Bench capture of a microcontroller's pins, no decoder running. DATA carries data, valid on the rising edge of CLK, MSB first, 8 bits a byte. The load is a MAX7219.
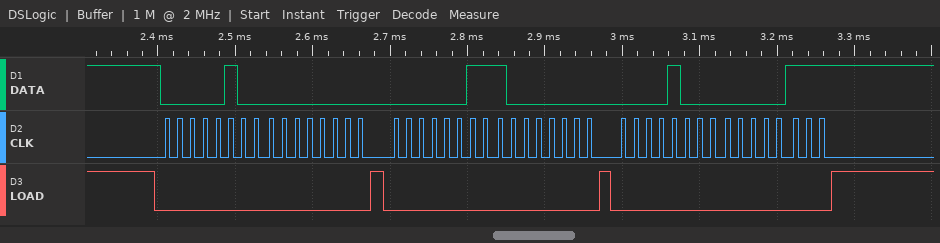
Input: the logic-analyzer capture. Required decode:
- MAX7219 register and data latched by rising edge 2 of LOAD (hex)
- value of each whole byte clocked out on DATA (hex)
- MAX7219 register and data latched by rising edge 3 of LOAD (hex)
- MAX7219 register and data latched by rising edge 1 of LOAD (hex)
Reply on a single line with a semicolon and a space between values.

register 0x3, data 0x80; 04 00 03 80 08 07; register 0x8, data 0x07; register 0x4, data 0x00
